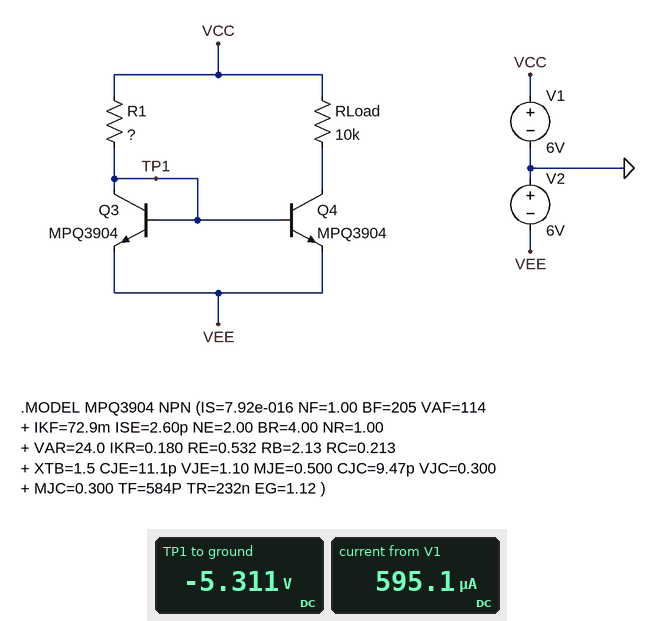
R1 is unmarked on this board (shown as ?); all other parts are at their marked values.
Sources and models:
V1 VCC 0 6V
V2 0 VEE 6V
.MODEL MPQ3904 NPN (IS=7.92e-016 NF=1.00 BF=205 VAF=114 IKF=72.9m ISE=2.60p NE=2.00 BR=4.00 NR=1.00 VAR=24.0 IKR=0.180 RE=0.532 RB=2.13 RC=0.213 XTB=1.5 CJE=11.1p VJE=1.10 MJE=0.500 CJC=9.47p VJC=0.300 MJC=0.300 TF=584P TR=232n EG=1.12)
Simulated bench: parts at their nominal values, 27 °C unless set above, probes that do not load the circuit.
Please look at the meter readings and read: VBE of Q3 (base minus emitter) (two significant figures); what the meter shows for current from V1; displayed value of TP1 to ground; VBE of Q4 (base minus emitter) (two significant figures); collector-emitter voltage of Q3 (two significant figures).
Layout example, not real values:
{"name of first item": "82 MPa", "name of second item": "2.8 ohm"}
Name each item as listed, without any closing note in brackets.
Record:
{"VBE of Q3 (base minus emitter)": "690 mV", "what the meter shows for current from V1": "595.1 µA", "displayed value of TP1 to ground": "-5.311 V", "VBE of Q4 (base minus emitter)": "690 mV", "collector-emitter voltage of Q3": "690 mV"}
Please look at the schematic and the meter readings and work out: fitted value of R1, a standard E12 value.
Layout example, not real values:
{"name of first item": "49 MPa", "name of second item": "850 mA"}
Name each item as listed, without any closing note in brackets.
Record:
{"fitted value of R1, a standard E12 value": "39 kΩ"}
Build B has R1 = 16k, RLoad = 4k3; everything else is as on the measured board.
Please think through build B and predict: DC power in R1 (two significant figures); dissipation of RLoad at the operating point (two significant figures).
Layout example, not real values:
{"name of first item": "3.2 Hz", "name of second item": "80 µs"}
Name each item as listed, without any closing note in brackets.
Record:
{"DC power in R1": "8.0 mW", "dissipation of RLoad at the operating point": "2.4 mW"}
